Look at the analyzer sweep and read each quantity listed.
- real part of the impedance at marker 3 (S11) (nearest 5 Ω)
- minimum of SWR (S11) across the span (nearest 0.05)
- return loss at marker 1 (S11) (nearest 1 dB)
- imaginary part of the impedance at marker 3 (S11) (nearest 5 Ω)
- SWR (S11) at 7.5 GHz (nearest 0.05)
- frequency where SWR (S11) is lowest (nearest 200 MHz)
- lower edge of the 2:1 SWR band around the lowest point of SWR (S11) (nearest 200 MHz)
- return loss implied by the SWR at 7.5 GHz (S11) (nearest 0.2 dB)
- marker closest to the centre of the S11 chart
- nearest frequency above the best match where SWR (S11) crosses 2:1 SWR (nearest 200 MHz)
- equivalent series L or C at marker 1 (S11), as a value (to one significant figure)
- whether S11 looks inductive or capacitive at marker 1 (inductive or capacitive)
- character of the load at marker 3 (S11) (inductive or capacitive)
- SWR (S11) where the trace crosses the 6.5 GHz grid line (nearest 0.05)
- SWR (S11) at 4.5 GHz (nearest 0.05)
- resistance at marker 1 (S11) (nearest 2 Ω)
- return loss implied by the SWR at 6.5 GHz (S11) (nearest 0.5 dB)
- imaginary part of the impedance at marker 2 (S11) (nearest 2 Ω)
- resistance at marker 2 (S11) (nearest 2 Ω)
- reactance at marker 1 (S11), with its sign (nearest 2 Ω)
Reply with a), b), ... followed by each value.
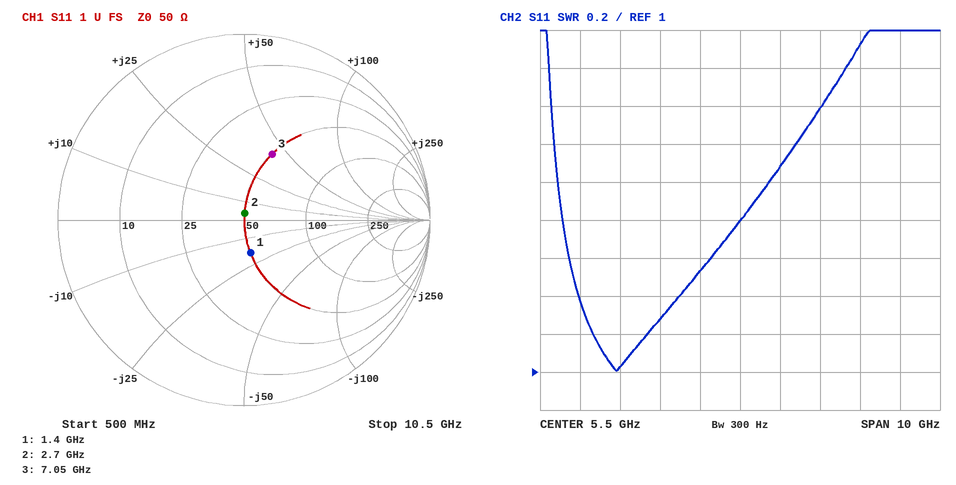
a) 50 Ω
b) 1.00
c) 15 dB
d) +40 Ω
e) 2.40
f) 2.4 GHz
g) 1.0 GHz
h) 7.8 dB
i) marker 2
j) 6.2 GHz
k) 6 pF
l) capacitive
m) inductive
n) 2.10
o) 1.55
p) 50 Ω
q) 9.0 dB
r) +4 Ω
s) 50 Ω
t) -18 Ω
